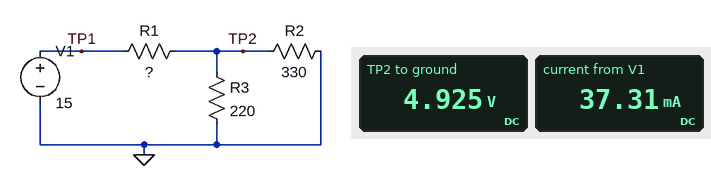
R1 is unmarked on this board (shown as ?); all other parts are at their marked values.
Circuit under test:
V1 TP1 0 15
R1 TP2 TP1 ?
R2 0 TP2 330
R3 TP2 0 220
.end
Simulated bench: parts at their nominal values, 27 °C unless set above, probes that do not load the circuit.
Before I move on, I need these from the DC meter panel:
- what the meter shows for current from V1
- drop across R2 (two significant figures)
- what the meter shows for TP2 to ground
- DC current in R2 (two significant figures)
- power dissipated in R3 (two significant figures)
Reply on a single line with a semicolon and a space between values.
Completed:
37.31 mA; 4.9 V; 4.925 V; 15 mA; 110 mW
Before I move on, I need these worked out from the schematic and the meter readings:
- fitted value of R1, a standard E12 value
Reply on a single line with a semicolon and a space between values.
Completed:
270 Ω
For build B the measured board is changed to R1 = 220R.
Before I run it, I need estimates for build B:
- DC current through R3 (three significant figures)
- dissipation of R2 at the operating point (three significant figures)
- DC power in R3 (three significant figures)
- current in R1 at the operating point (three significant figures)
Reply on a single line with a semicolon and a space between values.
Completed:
25.6 mA; 95.9 mW; 144 mW; 42.6 mA
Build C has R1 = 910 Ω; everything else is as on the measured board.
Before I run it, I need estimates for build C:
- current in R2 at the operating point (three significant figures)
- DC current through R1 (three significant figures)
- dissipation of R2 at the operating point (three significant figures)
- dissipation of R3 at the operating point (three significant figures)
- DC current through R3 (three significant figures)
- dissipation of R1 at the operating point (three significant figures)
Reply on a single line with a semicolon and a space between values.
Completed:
5.76 mA; 14.4 mA; 10.9 mW; 16.4 mW; 8.64 mA; 189 mW
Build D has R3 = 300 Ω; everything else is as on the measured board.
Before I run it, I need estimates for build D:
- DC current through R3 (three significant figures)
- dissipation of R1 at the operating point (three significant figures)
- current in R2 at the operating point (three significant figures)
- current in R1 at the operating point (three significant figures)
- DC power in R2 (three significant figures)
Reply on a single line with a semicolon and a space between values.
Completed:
18.4 mA; 333 mW; 16.7 mA; 35.1 mA; 92.3 mW
